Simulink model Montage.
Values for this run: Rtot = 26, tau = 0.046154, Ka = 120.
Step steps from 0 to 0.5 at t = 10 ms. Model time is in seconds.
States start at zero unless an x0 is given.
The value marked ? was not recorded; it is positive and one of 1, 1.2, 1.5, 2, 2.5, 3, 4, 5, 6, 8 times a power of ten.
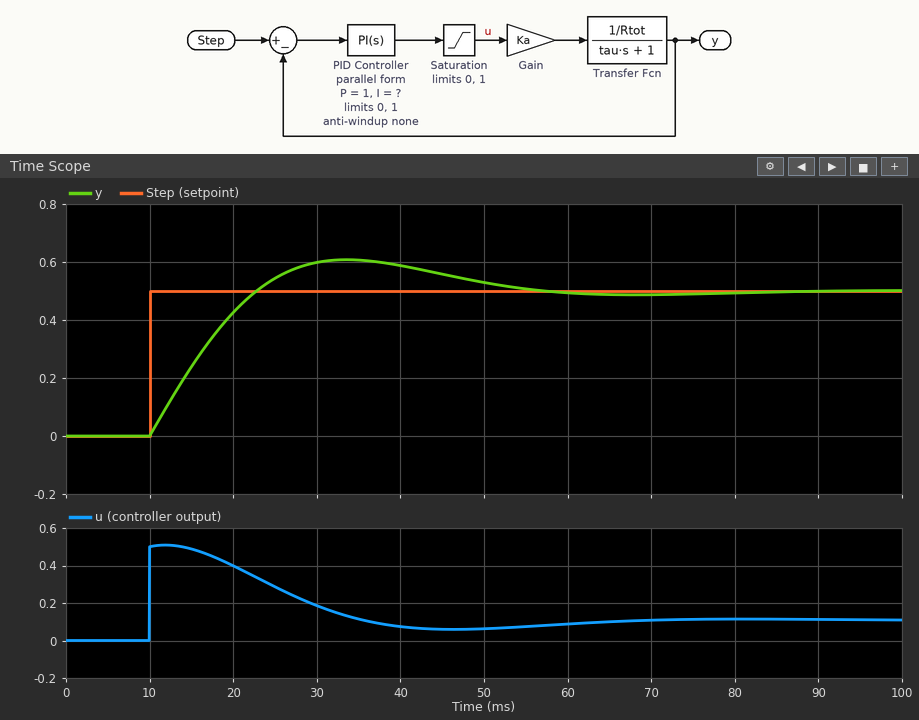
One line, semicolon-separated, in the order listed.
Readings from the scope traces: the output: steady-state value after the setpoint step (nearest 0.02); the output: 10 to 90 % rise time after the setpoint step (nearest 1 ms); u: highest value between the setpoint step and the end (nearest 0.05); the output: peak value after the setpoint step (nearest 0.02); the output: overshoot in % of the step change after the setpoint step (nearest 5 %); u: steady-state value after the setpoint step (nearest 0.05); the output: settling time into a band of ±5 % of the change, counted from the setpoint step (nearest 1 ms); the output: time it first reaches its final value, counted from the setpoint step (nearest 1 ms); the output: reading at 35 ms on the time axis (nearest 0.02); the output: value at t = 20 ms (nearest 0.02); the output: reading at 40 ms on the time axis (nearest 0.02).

0.50; 10 ms; 0.50; 0.60; 20 %; 0.10; 41 ms; 13 ms; 0.60; 0.42; 0.58
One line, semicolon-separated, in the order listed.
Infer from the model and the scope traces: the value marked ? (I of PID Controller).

120
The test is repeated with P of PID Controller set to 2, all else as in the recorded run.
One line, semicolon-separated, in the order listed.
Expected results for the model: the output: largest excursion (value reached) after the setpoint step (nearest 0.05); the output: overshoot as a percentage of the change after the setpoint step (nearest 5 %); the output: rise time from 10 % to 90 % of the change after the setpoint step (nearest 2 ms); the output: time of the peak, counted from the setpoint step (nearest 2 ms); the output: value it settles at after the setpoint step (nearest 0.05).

0.55; 10 %; 8 ms; 20 ms; 0.50
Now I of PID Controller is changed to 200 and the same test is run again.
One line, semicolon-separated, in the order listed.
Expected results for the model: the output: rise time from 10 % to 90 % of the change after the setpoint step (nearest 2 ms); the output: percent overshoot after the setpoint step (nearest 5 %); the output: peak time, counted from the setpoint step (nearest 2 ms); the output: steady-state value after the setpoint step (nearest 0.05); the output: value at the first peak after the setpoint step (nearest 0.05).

8 ms; 30 %; 18 ms; 0.50; 0.65
